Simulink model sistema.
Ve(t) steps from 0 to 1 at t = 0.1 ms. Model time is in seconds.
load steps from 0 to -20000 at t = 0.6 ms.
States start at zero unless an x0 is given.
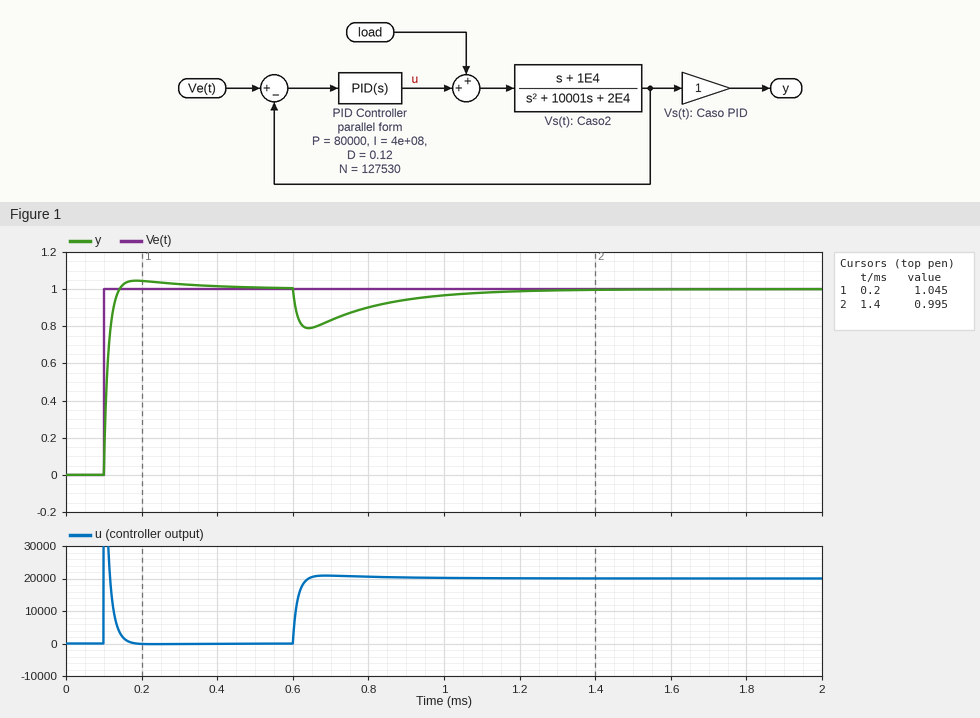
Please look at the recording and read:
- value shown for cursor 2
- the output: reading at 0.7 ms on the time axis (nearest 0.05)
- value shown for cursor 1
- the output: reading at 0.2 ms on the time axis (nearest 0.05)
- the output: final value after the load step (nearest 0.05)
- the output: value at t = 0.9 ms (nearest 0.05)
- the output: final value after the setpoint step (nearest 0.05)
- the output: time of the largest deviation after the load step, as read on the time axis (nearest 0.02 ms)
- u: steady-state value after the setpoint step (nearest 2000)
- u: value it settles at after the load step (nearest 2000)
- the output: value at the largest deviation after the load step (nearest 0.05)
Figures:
0.995
0.85
1.045
1.05
1.00
0.95
1.00
0.64 ms
0
20000
0.80
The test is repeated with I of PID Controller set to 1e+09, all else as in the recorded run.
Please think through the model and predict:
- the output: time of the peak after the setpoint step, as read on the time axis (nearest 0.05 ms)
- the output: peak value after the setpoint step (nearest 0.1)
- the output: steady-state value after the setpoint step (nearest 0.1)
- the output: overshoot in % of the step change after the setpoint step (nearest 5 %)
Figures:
0.15 ms
1.1
1.0
10 %
